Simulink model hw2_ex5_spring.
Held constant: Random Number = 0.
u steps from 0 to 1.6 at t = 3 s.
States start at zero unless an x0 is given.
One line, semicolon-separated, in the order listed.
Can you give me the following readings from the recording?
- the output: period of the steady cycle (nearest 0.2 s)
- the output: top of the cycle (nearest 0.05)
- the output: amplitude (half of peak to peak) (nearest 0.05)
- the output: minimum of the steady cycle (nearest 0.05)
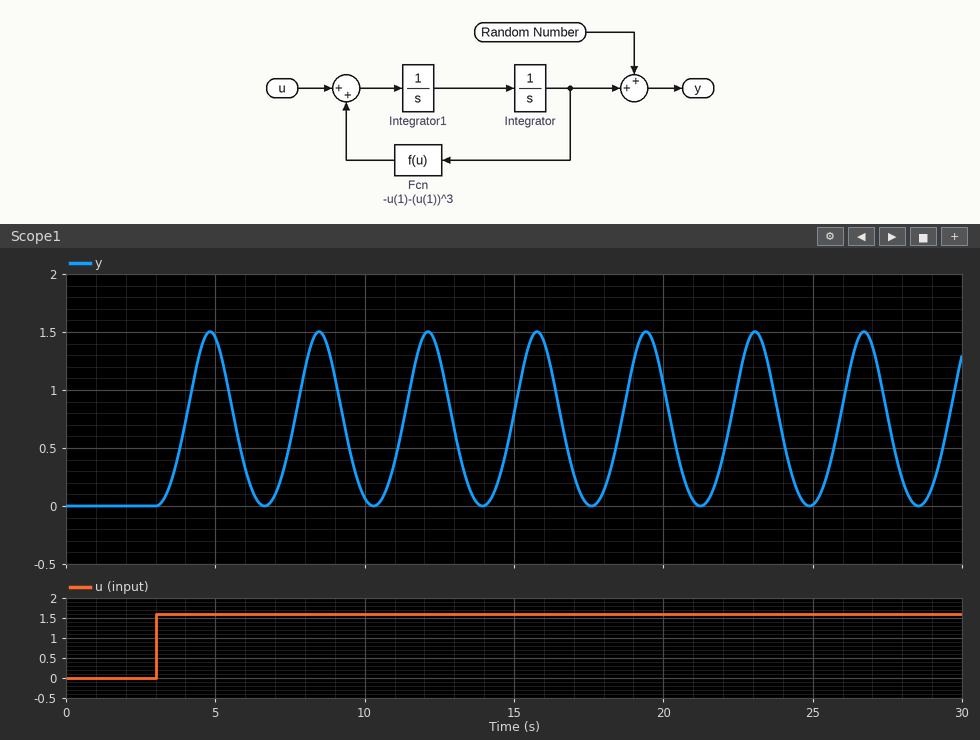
3.6 s; 1.50; 0.75; 0.00
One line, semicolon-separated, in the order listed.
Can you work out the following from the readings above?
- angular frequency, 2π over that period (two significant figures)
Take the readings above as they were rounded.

1.7 rad/s
